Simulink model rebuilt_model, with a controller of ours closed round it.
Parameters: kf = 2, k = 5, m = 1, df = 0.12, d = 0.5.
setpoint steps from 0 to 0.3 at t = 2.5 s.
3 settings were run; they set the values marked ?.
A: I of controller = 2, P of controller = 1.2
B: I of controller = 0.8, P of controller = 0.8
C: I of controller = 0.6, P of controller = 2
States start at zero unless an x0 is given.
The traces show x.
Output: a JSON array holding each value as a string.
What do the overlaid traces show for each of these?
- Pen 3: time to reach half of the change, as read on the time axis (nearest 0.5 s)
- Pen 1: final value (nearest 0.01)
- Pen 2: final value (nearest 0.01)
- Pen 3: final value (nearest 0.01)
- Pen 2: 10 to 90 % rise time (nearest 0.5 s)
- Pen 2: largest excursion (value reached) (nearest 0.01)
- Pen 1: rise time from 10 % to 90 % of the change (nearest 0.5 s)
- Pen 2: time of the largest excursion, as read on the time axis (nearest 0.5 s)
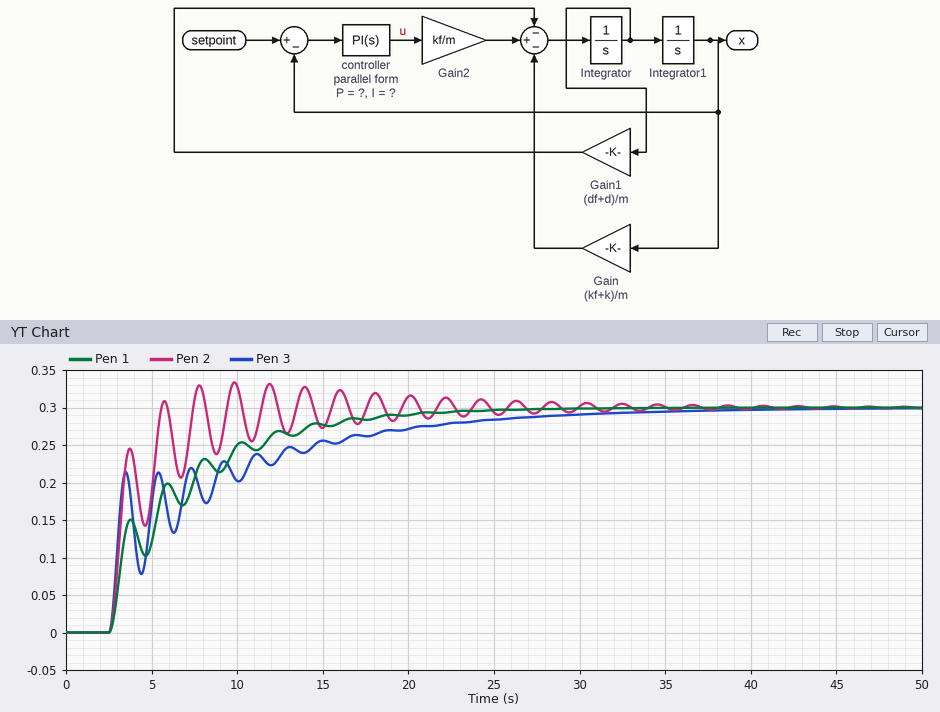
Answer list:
["3.0 s", "0.30", "0.30", "0.30", "2.5 s", "0.33", "11.0 s", "10.0 s"]
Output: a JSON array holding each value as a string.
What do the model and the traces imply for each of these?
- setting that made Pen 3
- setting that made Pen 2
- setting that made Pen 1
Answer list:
["C", "A", "B"]
